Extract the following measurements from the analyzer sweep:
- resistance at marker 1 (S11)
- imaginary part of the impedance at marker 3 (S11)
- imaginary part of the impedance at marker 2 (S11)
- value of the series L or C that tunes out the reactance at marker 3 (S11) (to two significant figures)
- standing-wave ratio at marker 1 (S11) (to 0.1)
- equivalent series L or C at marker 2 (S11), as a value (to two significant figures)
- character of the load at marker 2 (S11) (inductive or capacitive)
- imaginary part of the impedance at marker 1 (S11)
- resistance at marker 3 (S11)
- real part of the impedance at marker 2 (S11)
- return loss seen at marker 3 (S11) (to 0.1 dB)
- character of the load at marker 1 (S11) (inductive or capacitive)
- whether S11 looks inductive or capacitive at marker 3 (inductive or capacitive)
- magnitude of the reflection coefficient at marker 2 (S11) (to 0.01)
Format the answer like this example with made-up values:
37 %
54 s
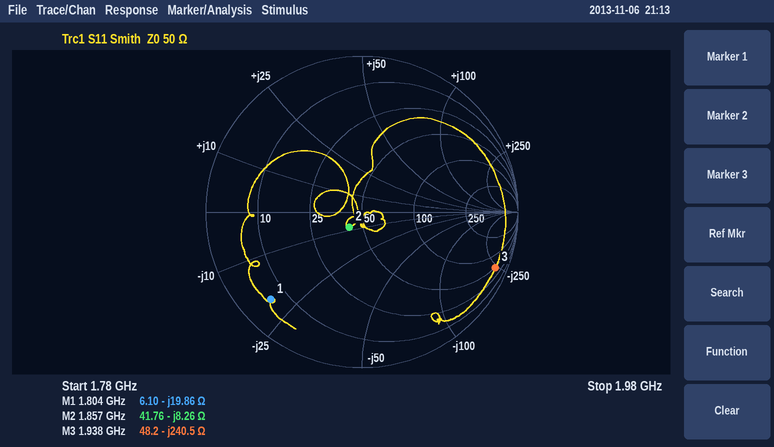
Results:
6.10 Ω
-240.5 Ω
-8.26 Ω
20 nH
9.5
10 pF
capacitive
-19.86 Ω
48.2 Ω
41.76 Ω
0.7 dB
capacitive
capacitive
0.13
